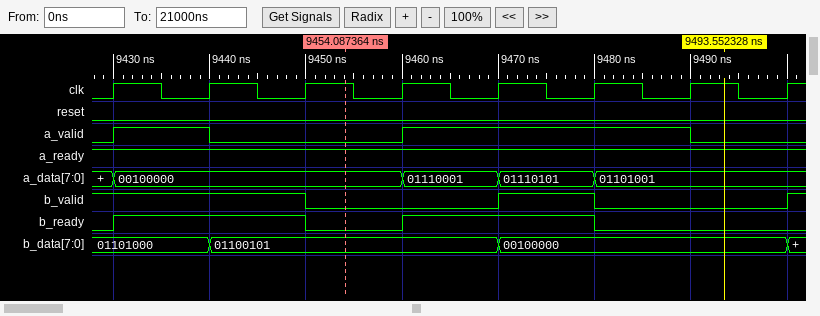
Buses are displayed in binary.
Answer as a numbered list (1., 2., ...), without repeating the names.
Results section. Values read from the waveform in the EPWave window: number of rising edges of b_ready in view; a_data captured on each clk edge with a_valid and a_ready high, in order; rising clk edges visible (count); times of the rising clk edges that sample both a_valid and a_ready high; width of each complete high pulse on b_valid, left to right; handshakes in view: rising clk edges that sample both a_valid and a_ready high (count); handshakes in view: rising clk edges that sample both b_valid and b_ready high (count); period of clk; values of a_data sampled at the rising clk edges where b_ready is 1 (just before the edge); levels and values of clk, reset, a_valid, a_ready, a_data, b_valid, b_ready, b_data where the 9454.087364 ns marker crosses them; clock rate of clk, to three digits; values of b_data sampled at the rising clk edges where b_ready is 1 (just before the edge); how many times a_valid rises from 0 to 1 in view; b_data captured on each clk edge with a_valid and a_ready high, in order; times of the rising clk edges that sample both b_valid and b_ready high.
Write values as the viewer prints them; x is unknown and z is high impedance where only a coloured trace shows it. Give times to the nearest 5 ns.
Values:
1. 2
2. 00100000, 01110001, 01110101, 01101001
3. 8
4. 9440 ns, 9470 ns, 9480 ns, 9490 ns
5. 10 ns
6. 4
7. 3
8. 10 ns
9. 00100000, 00100000, 01110001, 01110101
10. clk=1, reset=0, a_valid=0, a_ready=1, a_data=00100000, b_valid=0, b_ready=0, b_data=01100101
11. 100 MHz
12. 01101000, 01100101, 01100101, 00100000
13. 2
14. 01101000, 01100101, 00100000, 00100000
15. 9440 ns, 9450 ns, 9480 ns
